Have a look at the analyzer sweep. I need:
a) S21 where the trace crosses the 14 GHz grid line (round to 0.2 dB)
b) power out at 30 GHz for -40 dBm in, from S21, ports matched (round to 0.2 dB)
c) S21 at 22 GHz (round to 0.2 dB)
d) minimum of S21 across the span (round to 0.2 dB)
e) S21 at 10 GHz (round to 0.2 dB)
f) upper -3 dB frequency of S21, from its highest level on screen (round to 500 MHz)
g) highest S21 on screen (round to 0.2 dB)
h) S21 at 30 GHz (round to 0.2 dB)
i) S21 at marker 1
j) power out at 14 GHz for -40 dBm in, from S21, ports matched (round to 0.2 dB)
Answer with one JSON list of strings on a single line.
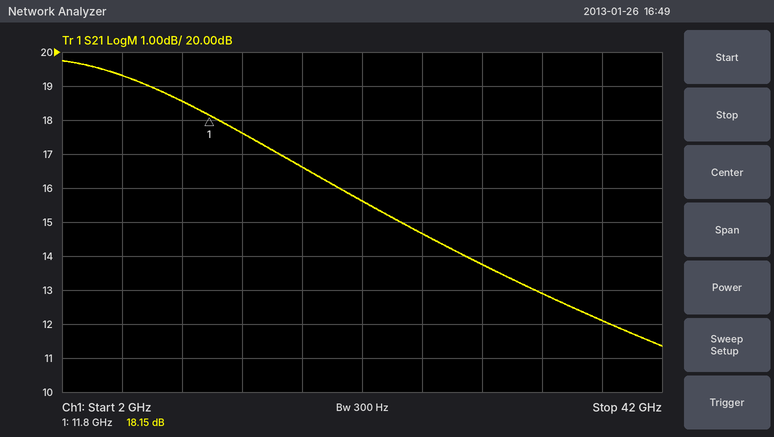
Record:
["17.6 dB", "-26.2 dBm", "15.6 dB", "11.4 dB", "18.6 dB", "17.5 GHz", "19.8 dB", "13.8 dB", "18.15 dB", "-22.4 dBm"]
